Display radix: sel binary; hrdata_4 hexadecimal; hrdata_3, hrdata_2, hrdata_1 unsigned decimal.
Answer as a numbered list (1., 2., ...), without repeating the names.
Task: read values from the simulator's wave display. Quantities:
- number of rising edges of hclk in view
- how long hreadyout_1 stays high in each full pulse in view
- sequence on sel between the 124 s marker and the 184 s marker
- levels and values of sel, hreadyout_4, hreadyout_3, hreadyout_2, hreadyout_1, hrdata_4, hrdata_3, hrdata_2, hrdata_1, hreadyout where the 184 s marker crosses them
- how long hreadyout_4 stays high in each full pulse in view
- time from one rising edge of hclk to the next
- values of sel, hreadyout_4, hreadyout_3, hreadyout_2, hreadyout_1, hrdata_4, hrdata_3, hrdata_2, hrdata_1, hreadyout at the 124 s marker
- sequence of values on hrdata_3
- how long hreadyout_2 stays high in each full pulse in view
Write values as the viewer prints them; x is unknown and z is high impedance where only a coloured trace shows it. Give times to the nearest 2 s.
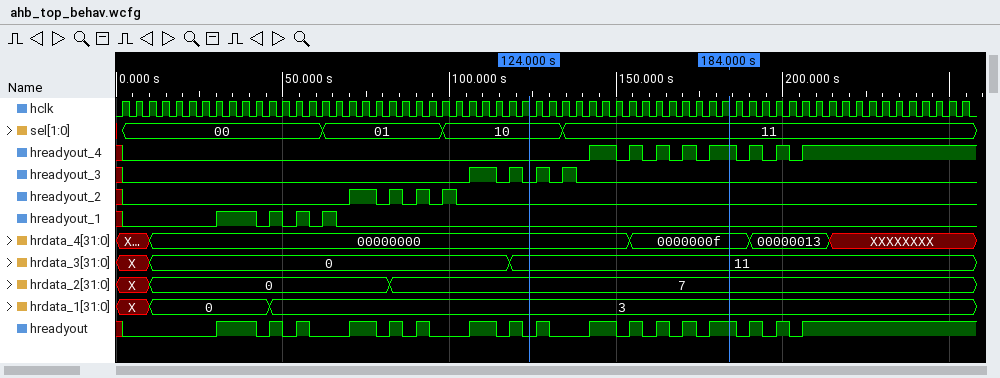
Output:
1. 64
2. 12 s, 4 s, 4 s, 4 s
3. 10, 11
4. sel=11, hreadyout_4=1, hreadyout_3=0, hreadyout_2=0, hreadyout_1=0, hrdata_4=0000000f, hrdata_3=11, hrdata_2=7, hrdata_1=3, hreadyout=1
5. 8 s, 4 s, 4 s, 4 s, 8 s, 4 s, 4 s
6. 4 s
7. sel=10, hreadyout_4=0, hreadyout_3=0, hreadyout_2=0, hreadyout_1=0, hrdata_4=00000000, hrdata_3=11, hrdata_2=7, hrdata_1=3, hreadyout=0
8. X, 0, 11
9. 8 s, 4 s, 4 s, 4 s
